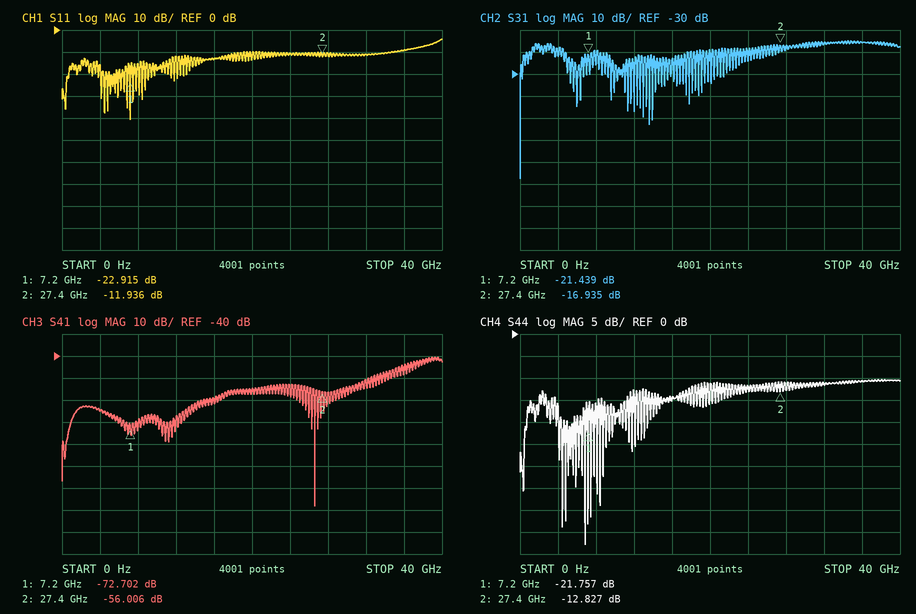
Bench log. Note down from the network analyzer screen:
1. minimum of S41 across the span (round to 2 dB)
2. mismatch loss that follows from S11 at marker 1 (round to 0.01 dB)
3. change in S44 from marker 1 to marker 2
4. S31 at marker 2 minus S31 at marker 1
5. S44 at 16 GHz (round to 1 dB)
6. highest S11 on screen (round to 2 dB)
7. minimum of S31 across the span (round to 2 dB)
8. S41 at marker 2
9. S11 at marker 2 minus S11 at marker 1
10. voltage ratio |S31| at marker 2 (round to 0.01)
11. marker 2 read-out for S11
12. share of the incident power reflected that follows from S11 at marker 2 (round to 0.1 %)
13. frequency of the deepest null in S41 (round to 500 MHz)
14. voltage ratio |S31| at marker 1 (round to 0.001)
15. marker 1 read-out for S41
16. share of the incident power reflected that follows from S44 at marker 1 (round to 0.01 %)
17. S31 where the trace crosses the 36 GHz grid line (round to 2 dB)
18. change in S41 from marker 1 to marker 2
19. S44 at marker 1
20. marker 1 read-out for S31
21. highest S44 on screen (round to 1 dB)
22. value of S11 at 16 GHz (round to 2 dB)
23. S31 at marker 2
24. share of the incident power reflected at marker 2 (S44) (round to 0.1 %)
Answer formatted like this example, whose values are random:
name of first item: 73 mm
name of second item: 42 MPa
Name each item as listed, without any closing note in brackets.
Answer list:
minimum of S41 across the span: -108 dB
mismatch loss that follows from S11 at marker 1: 0.02 dB
change in S44 from marker 1 to marker 2: 8.930 dB
S31 at marker 2 minus S31 at marker 1: 4.504 dB
S44 at 16 GHz: -15 dB
highest S11 on screen: -4 dB
minimum of S31 across the span: -78 dB
S41 at marker 2: -56.006 dB
S11 at marker 2 minus S11 at marker 1: 10.979 dB
voltage ratio |S31| at marker 2: 0.14
marker 2 read-out for S11: -11.936 dB
share of the incident power reflected that follows from S11 at marker 2: 6.4 %
frequency of the deepest null in S41: 26.5 GHz
voltage ratio |S31| at marker 1: 0.085
marker 1 read-out for S41: -72.702 dB
share of the incident power reflected that follows from S44 at marker 1: 0.67 %
S31 where the trace crosses the 36 GHz grid line: -16 dB
change in S41 from marker 1 to marker 2: 16.696 dB
S44 at marker 1: -21.757 dB
marker 1 read-out for S31: -21.439 dB
highest S44 on screen: -10 dB
value of S11 at 16 GHz: -14 dB
S31 at marker 2: -16.935 dB
share of the incident power reflected at marker 2 (S44): 5.2 %
